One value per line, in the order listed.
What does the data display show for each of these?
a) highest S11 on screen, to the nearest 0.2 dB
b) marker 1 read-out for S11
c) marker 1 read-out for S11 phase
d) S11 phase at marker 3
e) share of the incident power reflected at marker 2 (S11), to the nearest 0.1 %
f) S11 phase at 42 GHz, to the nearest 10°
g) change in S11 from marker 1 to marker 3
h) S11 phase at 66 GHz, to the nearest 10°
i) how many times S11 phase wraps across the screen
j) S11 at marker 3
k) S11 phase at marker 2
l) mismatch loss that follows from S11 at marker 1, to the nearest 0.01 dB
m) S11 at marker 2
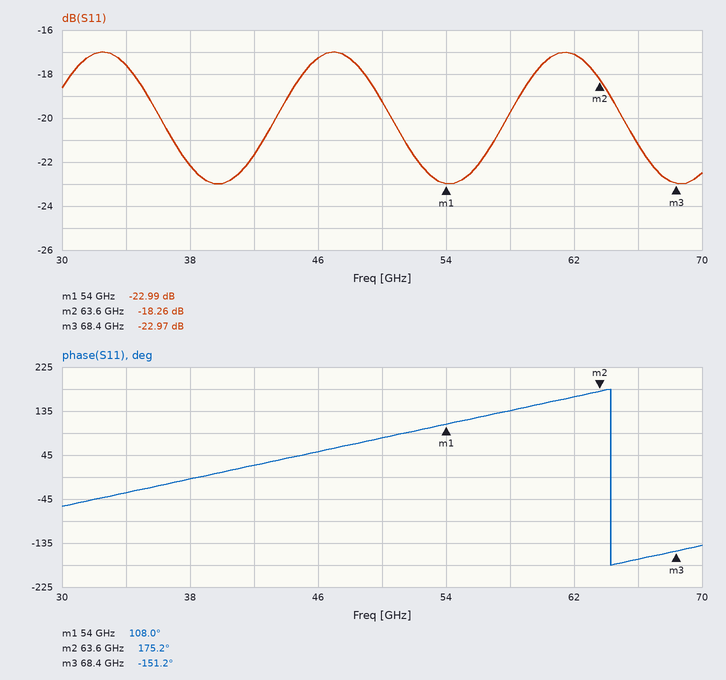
-17.0 dB
-22.99 dB
108.0°
-151.2°
1.5 %
20°
0.02 dB
-170°
1
-22.97 dB
175.2°
0.02 dB
-18.26 dB
